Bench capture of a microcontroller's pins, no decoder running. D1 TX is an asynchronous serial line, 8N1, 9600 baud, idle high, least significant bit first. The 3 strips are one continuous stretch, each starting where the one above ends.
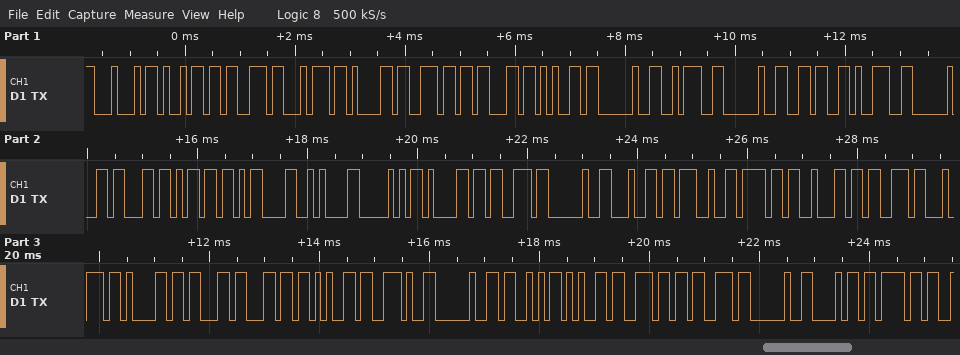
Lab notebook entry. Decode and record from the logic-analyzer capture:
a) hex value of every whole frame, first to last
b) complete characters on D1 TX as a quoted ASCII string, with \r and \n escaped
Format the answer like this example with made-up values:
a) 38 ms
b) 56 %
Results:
a) 44 69 73 74 61 6E 63 65 20 3A 20 36 39 20 63 6D 0D 0A 50 61 73 20 64 27 6F 62 73 74 61 63 6C 65 2E 20 53 65 6E 73 20 68 6F
b) "Distance : 69 cm\r\nPas d'obstacle. Sens ho"
